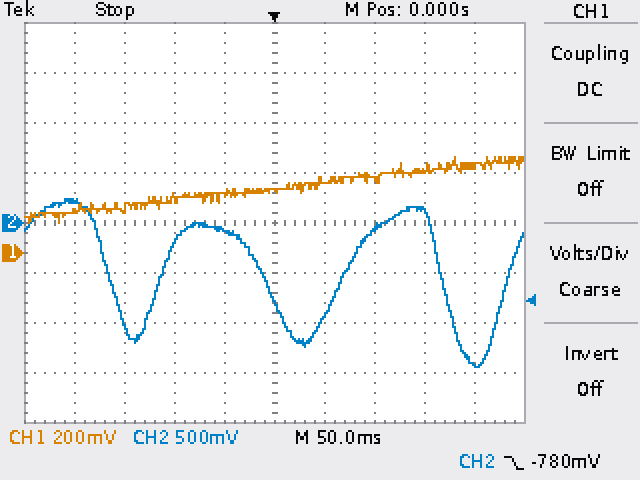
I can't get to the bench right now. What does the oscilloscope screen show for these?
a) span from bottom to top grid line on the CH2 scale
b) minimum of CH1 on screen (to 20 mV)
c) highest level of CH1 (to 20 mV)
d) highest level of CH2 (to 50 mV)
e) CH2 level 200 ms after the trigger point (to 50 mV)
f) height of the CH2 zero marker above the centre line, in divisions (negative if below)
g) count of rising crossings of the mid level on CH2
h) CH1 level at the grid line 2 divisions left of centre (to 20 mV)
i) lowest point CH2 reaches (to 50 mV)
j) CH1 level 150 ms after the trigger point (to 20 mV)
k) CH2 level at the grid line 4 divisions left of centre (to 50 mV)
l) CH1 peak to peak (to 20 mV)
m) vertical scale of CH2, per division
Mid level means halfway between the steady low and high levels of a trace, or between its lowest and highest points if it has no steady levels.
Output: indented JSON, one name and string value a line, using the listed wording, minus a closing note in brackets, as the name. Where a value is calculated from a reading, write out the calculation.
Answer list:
{
  "span from bottom to top grid line on the CH2 scale": "4 V",
  "minimum of CH1 on screen": "120 mV",
  "highest level of CH1": "380 mV",
  "highest level of CH2": "250 mV",
  "CH2 level 200 ms after the trigger point": "-1.40 V",
  "height of the CH2 zero marker above the centre line, in divisions": "0.0 div",
  "count of rising crossings of the mid level on CH2": "3",
  "CH1 level at the grid line 2 divisions left of centre": "220 mV",
  "lowest point CH2 reaches": "-1.45 V",
  "CH1 level 150 ms after the trigger point": "340 mV",
  "CH2 level at the grid line 4 divisions left of centre": "200 mV",
  "CH1 peak to peak": "380 mV − (120 mV) = 260 mV",
  "vertical scale of CH2, per division": "500 mV"
}
